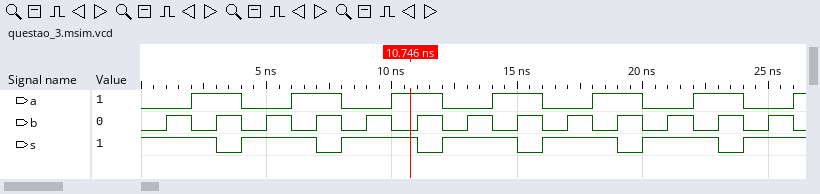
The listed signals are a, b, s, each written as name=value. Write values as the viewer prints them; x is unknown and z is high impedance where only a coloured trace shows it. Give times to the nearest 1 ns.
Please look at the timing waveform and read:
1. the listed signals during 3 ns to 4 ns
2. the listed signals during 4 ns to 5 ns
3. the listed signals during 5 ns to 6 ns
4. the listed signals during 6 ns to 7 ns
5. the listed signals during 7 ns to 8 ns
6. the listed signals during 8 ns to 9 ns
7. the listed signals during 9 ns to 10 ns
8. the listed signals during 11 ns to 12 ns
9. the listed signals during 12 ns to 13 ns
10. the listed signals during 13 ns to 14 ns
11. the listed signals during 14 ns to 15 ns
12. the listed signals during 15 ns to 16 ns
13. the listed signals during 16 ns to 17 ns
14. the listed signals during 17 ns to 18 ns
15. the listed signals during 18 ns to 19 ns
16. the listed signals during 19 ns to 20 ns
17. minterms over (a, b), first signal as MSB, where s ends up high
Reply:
a=1, b=1, s=0
a=0, b=0, s=1
a=0, b=1, s=1
a=1, b=0, s=1
a=1, b=1, s=0
a=0, b=0, s=1
a=0, b=1, s=1
a=1, b=1, s=0
a=0, b=0, s=1
a=0, b=1, s=1
a=1, b=0, s=1
a=1, b=1, s=0
a=0, b=0, s=1
a=0, b=1, s=1
a=1, b=0, s=1
a=1, b=1, s=0
0, 1, 2
